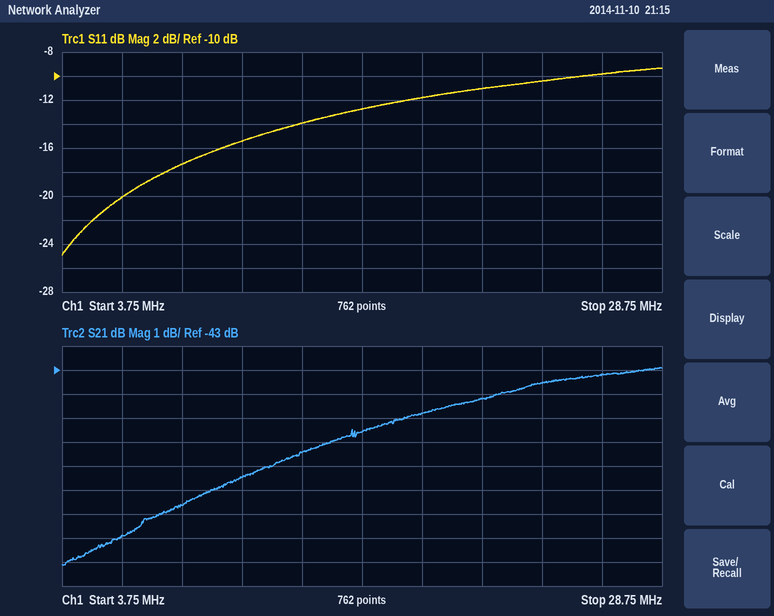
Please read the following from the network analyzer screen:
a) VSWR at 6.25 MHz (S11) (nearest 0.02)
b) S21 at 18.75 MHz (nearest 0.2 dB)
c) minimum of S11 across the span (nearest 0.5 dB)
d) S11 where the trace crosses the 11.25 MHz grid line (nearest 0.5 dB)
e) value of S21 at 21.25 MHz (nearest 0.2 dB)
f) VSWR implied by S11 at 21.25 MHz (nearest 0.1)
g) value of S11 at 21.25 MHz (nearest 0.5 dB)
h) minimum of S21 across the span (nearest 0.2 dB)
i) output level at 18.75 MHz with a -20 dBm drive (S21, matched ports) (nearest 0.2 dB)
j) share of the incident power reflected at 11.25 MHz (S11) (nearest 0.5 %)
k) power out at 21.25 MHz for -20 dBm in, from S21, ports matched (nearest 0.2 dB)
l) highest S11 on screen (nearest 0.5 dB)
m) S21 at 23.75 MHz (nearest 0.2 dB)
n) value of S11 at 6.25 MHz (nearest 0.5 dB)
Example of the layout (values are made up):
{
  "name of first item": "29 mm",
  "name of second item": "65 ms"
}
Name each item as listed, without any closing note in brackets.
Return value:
{
  "VSWR at 6.25 MHz (S11)": "1.22",
  "S21 at 18.75 MHz": "-44.8 dB",
  "minimum of S11 across the span": "-25.0 dB",
  "S11 where the trace crosses the 11.25 MHz grid line": "-15.5 dB",
  "value of S21 at 21.25 MHz": "-44.2 dB",
  "VSWR implied by S11 at 21.25 MHz": "1.8",
  "value of S11 at 21.25 MHz": "-11.0 dB",
  "minimum of S21 across the span": "-51.2 dB",
  "output level at 18.75 MHz with a -20 dBm drive (S21, matched ports)": "-64.8 dBm",
  "share of the incident power reflected at 11.25 MHz (S11)": "3.0 %",
  "power out at 21.25 MHz for -20 dBm in, from S21, ports matched": "-64.2 dBm",
  "highest S11 on screen": "-9.5 dB",
  "S21 at 23.75 MHz": "-43.6 dB",
  "value of S11 at 6.25 MHz": "-20.0 dB"
}
